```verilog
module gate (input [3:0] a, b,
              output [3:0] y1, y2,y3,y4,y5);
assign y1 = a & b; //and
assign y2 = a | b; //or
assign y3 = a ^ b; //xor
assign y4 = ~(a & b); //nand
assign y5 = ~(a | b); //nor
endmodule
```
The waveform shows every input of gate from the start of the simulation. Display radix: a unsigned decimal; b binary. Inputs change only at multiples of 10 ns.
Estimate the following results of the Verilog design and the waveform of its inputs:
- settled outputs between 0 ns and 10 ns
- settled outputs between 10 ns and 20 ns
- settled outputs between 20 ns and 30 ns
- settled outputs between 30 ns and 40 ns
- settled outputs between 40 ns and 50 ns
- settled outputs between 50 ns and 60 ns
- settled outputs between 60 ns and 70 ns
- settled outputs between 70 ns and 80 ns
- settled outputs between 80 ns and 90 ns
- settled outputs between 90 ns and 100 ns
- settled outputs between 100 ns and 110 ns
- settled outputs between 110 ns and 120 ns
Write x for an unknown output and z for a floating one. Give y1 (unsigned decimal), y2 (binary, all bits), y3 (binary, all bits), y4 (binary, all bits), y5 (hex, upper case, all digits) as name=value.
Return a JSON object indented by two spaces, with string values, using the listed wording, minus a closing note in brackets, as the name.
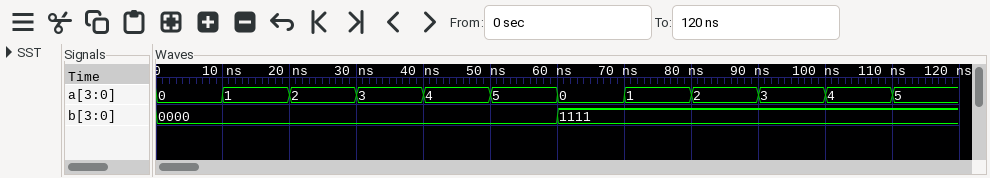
{
  "settled outputs between 0 ns and 10 ns": "y1=0, y2=0000, y3=0000, y4=1111, y5=F",
  "settled outputs between 10 ns and 20 ns": "y1=0, y2=0001, y3=0001, y4=1111, y5=E",
  "settled outputs between 20 ns and 30 ns": "y1=0, y2=0010, y3=0010, y4=1111, y5=D",
  "settled outputs between 30 ns and 40 ns": "y1=0, y2=0011, y3=0011, y4=1111, y5=C",
  "settled outputs between 40 ns and 50 ns": "y1=0, y2=0100, y3=0100, y4=1111, y5=B",
  "settled outputs between 50 ns and 60 ns": "y1=0, y2=0101, y3=0101, y4=1111, y5=A",
  "settled outputs between 60 ns and 70 ns": "y1=0, y2=1111, y3=1111, y4=1111, y5=0",
  "settled outputs between 70 ns and 80 ns": "y1=1, y2=1111, y3=1110, y4=1110, y5=0",
  "settled outputs between 80 ns and 90 ns": "y1=2, y2=1111, y3=1101, y4=1101, y5=0",
  "settled outputs between 90 ns and 100 ns": "y1=3, y2=1111, y3=1100, y4=1100, y5=0",
  "settled outputs between 100 ns and 110 ns": "y1=4, y2=1111, y3=1011, y4=1011, y5=0",
  "settled outputs between 110 ns and 120 ns": "y1=5, y2=1111, y3=1010, y4=1010, y5=0"
}
